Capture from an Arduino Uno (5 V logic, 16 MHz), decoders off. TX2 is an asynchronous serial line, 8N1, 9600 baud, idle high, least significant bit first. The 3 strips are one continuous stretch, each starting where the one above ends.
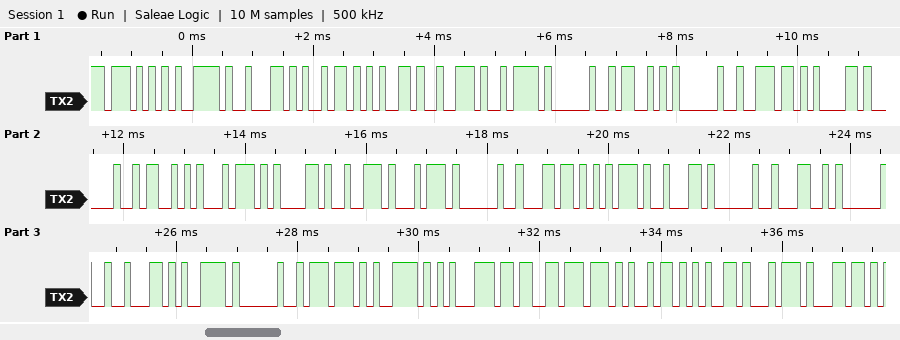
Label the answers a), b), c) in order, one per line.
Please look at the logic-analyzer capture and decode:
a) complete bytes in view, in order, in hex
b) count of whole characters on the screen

a) 57 79 62 69 65 72 7A 20 53 20 6E 61 20 53 74 61 72 74 20 6C 75 62 20 4C 20 62 79 20 77 79 C5 9B 77 69 65 74 6C
b) 37
